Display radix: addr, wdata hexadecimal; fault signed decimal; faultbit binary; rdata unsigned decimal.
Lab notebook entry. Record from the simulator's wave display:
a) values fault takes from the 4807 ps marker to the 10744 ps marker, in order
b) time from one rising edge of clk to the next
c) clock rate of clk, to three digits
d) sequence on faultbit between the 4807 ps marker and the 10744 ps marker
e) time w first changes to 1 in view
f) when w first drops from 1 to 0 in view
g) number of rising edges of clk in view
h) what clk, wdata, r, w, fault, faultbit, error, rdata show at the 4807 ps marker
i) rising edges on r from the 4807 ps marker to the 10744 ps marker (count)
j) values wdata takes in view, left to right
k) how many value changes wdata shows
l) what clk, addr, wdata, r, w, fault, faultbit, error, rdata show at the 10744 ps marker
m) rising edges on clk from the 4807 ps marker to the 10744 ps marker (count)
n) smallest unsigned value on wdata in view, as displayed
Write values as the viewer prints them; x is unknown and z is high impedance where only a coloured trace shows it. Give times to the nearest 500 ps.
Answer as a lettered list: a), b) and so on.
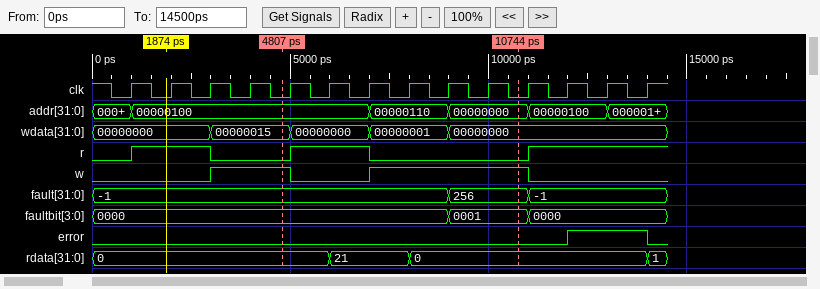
a) -1, 256
b) 1000 ps
c) 1.00 GHz
d) 0000, 0001
e) 3000 ps
f) 5000 ps
g) 14
h) clk=0, wdata=00000015, r=0, w=1, fault=-1, faultbit=0000, error=0, rdata=0
i) 1
j) 00000000, 00000015, 00000000, 00000001, 00000000
k) 4
l) clk=0, addr=00000000, wdata=00000000, r=0, w=1, fault=256, faultbit=0001, error=0, rdata=0
m) 6
n) 00000000
